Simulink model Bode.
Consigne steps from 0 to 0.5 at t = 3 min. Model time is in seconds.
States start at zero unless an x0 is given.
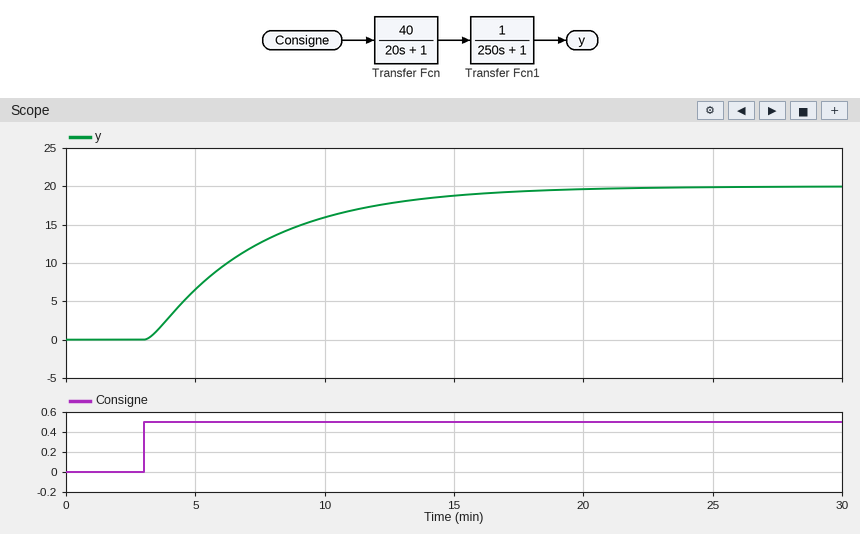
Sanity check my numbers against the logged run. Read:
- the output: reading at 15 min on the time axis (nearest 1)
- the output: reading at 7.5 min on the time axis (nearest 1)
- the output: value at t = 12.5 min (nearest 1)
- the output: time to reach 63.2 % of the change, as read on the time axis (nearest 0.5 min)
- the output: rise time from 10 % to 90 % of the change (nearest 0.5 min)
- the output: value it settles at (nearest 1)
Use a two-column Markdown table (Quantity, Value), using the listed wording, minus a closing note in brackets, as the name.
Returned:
| Quantity | Value |
|---|---|
| the output: reading at 15 min on the time axis | 19 |
| the output: reading at 7.5 min on the time axis | 13 |
| the output: value at t = 12.5 min | 18 |
| the output: time to reach 63.2 % of the change, as read on the time axis | 7.5 min |
| the output: rise time from 10 % to 90 % of the change | 9.0 min |
| the output: value it settles at | 20 |
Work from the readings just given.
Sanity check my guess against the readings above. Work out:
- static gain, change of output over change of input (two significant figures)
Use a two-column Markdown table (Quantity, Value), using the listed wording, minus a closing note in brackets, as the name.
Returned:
| Quantity | Value |
|---|---|
| static gain, change of output over change of input | 40 |
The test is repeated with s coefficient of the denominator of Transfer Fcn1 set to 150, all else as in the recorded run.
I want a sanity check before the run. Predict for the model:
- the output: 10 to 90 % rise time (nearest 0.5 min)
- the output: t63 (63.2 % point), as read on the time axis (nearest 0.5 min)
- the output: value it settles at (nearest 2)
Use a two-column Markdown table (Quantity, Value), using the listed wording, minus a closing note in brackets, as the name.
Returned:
| Quantity | Value |
|---|---|
| the output: 10 to 90 % rise time | 5.5 min |
| the output: t63 (63.2 % point), as read on the time axis | 6.0 min |
| the output: value it settles at | 20 |
